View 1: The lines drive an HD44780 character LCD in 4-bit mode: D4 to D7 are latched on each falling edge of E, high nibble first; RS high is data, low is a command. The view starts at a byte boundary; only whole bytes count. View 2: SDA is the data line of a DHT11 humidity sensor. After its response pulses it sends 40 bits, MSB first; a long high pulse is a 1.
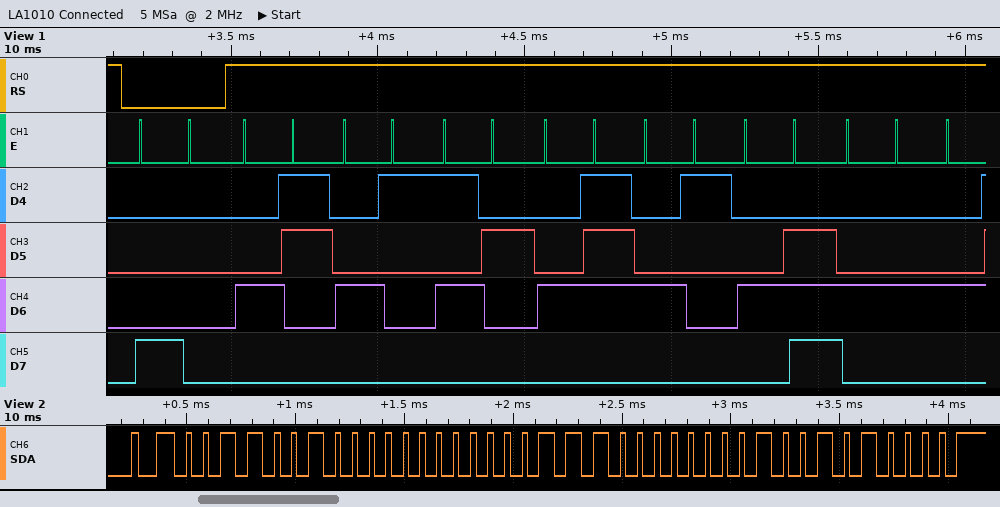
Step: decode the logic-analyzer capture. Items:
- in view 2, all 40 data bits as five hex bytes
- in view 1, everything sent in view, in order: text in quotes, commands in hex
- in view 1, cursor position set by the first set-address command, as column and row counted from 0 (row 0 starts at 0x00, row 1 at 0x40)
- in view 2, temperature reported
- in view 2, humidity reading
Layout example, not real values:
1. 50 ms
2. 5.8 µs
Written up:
1. 32 00 1C 02 50
2. 0x80 "CARGAND"
3. column 0, row 0
4. 28.2 °C
5. 50 %
